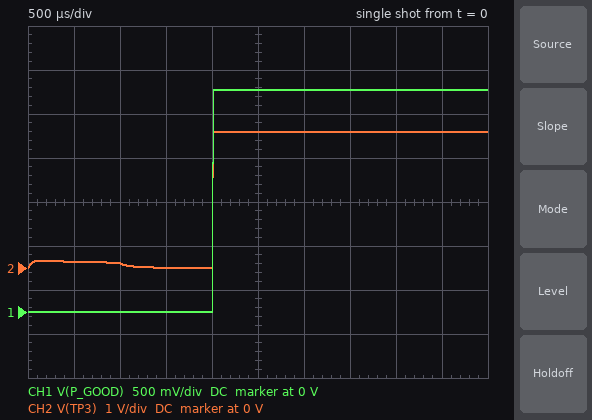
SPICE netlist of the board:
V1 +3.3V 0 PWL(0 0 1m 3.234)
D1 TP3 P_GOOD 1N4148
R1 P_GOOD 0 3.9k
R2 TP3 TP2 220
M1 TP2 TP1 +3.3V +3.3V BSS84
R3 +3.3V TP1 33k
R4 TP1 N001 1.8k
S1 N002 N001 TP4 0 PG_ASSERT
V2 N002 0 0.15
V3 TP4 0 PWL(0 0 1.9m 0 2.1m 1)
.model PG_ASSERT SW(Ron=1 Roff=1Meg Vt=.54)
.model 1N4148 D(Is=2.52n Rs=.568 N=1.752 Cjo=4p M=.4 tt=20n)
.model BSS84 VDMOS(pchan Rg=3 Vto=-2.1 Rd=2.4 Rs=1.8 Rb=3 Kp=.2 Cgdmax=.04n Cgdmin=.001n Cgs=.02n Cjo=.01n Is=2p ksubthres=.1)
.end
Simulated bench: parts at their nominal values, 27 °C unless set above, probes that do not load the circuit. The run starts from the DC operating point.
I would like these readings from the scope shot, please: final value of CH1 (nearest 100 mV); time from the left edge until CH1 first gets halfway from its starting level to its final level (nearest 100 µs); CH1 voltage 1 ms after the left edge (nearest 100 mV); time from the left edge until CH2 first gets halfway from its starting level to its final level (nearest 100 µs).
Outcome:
2.5 V
2.0 ms
0 V
2.0 ms
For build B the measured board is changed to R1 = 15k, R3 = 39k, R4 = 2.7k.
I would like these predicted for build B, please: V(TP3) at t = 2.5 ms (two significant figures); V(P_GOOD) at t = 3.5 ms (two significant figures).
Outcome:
3.2 V
2.7 V
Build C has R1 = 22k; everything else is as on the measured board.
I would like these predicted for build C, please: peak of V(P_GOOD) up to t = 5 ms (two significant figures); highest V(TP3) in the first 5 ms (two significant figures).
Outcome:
2.7 V
3.2 V
